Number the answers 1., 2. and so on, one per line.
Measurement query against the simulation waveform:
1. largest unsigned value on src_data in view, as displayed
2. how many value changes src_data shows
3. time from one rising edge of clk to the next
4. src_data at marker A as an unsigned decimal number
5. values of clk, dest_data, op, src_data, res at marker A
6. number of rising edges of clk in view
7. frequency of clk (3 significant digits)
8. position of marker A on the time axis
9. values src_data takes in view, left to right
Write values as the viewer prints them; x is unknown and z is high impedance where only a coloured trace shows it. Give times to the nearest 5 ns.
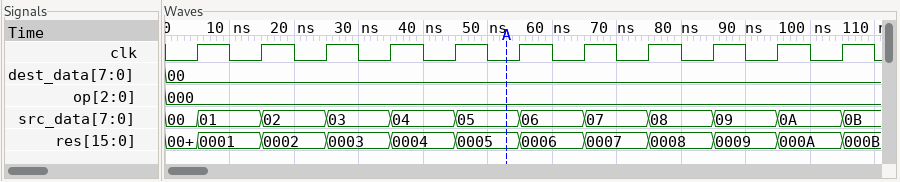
1. 0B
2. 11
3. 10 ns
4. 5
5. clk=0, dest_data=00, op=000, src_data=05, res=0005
6. 11
7. 100 MHz
8. 55 ns
9. 00, 01, 02, 03, 04, 05, 06, 07, 08, 09, 0A, 0B
